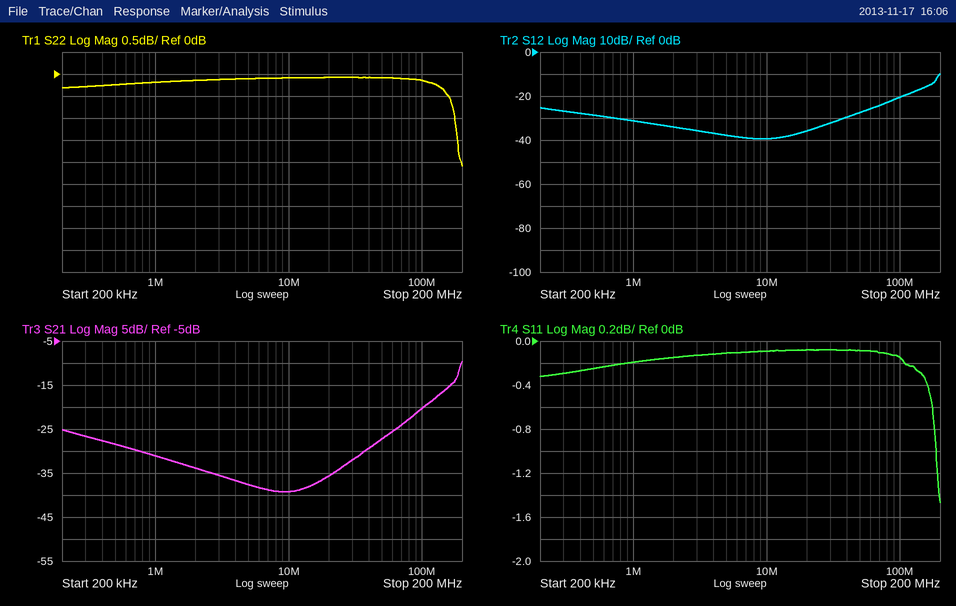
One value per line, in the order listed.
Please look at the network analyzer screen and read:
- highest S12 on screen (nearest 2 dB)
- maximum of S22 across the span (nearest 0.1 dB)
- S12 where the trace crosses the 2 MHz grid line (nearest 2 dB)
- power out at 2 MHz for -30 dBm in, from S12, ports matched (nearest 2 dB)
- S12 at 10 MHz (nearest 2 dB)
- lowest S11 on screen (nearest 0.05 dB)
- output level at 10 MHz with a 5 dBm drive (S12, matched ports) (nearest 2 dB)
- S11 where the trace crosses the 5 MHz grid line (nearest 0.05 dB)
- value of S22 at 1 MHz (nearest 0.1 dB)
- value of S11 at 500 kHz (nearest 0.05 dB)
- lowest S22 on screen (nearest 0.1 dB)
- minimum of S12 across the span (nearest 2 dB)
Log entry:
-10 dB
-0.1 dB
-34 dB
-64 dBm
-40 dB
-1.45 dB
-34 dBm
-0.10 dB
-0.2 dB
-0.25 dB
-2.1 dB
-40 dB
